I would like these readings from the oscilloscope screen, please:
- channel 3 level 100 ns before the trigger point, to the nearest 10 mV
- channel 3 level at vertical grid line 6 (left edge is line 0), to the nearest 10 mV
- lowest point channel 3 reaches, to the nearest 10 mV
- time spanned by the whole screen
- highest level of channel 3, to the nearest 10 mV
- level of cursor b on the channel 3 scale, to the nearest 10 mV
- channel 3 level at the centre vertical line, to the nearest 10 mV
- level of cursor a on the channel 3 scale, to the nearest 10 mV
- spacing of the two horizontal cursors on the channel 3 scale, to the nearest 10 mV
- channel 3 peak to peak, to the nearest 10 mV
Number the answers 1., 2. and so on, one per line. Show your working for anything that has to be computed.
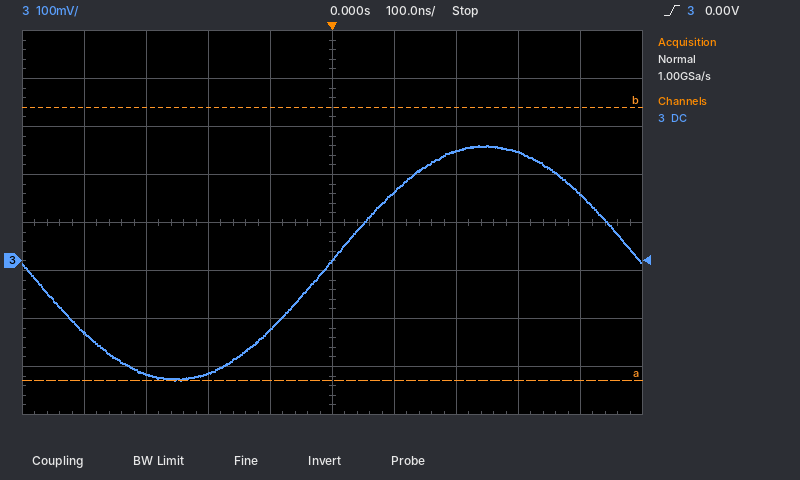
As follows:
1. -140 mV
2. 140 mV
3. -250 mV
4. 1 µs
5. 240 mV
6. 320 mV
7. 0 mV
8. -250 mV
9. 570 mV
10. 240 mV − (-250 mV) = 490 mV
